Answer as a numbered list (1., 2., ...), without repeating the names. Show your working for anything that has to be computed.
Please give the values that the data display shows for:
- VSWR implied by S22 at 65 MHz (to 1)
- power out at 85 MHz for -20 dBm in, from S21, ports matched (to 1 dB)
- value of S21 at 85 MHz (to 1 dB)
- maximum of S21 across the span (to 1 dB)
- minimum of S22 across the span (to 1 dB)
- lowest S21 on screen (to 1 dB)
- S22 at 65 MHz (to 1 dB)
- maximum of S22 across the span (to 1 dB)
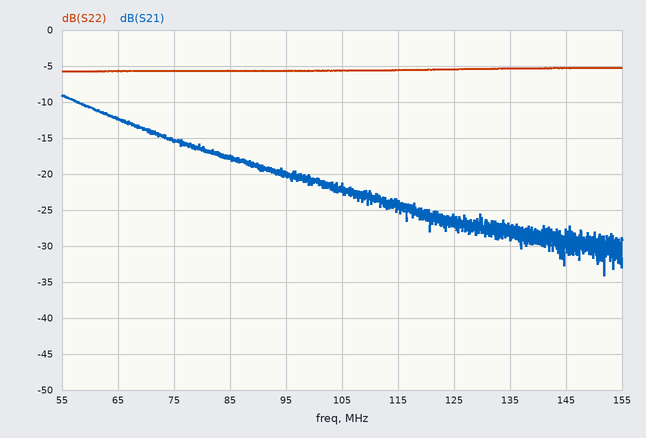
1. |Γ| = 10^(-6/20) = 0.5012; VSWR = (1 + 0.5012)/(1 − 0.5012) ≈ 3
2. -20 dBm + (-18 dB) = -38 dBm
3. -18 dB
4. -9 dB
5. -6 dB
6. -34 dB
7. -6 dB
8. -5 dB
